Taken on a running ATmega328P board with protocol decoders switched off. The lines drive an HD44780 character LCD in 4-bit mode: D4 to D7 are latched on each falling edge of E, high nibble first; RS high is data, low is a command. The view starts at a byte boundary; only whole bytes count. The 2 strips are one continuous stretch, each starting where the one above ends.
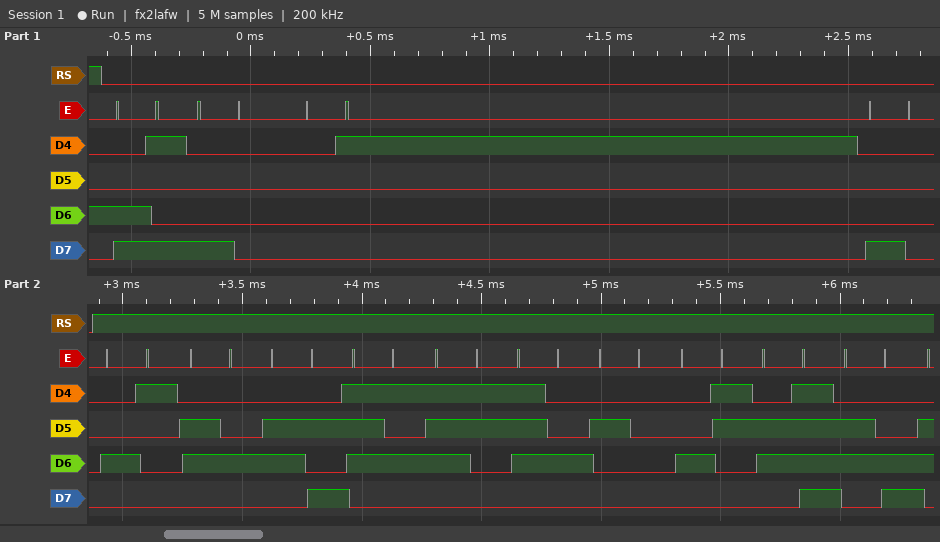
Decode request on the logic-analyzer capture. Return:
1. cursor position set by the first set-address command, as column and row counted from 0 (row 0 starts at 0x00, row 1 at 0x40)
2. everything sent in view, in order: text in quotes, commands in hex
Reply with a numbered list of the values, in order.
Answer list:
1. column 9, row 1
2. 0xC9 0x80 0x01 0x80 "Adjust Col"
